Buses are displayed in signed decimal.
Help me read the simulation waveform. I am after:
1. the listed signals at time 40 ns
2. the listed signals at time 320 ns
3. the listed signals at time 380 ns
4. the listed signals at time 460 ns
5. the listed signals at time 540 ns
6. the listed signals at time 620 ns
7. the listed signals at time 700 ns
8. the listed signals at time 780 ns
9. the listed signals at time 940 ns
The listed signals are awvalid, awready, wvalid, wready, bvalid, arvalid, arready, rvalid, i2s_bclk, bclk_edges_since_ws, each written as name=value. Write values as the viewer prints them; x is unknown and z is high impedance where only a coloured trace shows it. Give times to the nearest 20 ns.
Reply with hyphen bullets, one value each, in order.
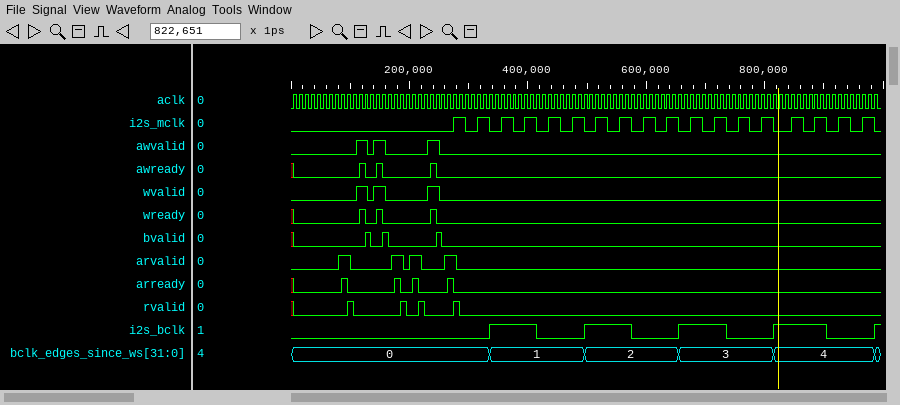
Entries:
- awvalid=0, awready=0, wvalid=0, wready=0, bvalid=0, arvalid=0, arready=0, rvalid=0, i2s_bclk=0, bclk_edges_since_ws=0
- awvalid=0, awready=0, wvalid=0, wready=0, bvalid=0, arvalid=0, arready=0, rvalid=0, i2s_bclk=0, bclk_edges_since_ws=0
- awvalid=0, awready=0, wvalid=0, wready=0, bvalid=0, arvalid=0, arready=0, rvalid=0, i2s_bclk=1, bclk_edges_since_ws=1
- awvalid=0, awready=0, wvalid=0, wready=0, bvalid=0, arvalid=0, arready=0, rvalid=0, i2s_bclk=0, bclk_edges_since_ws=1
- awvalid=0, awready=0, wvalid=0, wready=0, bvalid=0, arvalid=0, arready=0, rvalid=0, i2s_bclk=1, bclk_edges_since_ws=2
- awvalid=0, awready=0, wvalid=0, wready=0, bvalid=0, arvalid=0, arready=0, rvalid=0, i2s_bclk=0, bclk_edges_since_ws=2
- awvalid=0, awready=0, wvalid=0, wready=0, bvalid=0, arvalid=0, arready=0, rvalid=0, i2s_bclk=1, bclk_edges_since_ws=3
- awvalid=0, awready=0, wvalid=0, wready=0, bvalid=0, arvalid=0, arready=0, rvalid=0, i2s_bclk=0, bclk_edges_since_ws=3
- awvalid=0, awready=0, wvalid=0, wready=0, bvalid=0, arvalid=0, arready=0, rvalid=0, i2s_bclk=0, bclk_edges_since_ws=4
